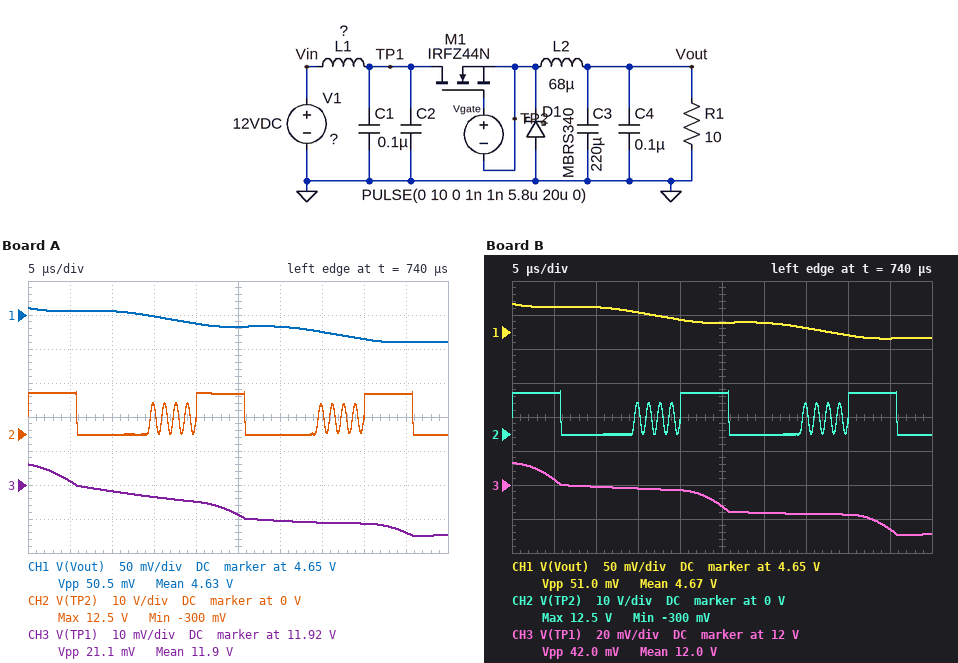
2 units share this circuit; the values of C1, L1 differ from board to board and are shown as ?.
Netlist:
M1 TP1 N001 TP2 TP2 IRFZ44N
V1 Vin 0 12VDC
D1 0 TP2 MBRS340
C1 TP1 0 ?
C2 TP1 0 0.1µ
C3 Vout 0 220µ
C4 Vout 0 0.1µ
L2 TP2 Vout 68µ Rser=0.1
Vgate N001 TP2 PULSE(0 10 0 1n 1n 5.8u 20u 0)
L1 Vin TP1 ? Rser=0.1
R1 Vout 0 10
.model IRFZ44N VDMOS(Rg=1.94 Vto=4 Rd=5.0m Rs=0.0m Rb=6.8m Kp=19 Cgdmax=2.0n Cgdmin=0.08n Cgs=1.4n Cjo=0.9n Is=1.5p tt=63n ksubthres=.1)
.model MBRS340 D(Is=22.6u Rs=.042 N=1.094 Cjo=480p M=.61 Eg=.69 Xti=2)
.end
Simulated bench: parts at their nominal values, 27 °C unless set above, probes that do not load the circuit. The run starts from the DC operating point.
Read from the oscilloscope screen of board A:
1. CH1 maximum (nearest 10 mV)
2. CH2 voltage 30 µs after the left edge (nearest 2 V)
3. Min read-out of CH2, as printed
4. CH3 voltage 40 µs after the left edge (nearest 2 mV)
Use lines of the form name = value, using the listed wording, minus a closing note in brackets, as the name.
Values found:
CH1 maximum = 4.66 V
CH2 voltage 30 µs after the left edge = 0 V
Min read-out of CH2, as printed = -300 mV
CH3 voltage 40 µs after the left edge = 11.908 V
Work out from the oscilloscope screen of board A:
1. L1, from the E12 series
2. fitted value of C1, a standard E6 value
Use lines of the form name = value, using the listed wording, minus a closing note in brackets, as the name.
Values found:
L1, from the E12 series = 18 µH
fitted value of C1, a standard E6 value = 470 µF
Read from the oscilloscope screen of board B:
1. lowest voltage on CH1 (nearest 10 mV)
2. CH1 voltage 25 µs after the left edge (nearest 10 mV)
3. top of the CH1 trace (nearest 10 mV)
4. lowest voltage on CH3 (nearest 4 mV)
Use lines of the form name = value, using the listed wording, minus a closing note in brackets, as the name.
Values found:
lowest voltage on CH1 = 4.64 V
CH1 voltage 25 µs after the left edge = 4.66 V
top of the CH1 trace = 4.69 V
lowest voltage on CH3 = 11.972 V
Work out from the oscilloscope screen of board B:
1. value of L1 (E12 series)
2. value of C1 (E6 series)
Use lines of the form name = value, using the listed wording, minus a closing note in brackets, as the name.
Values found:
value of L1 = 15 µH
value of C1 = 150 µF
